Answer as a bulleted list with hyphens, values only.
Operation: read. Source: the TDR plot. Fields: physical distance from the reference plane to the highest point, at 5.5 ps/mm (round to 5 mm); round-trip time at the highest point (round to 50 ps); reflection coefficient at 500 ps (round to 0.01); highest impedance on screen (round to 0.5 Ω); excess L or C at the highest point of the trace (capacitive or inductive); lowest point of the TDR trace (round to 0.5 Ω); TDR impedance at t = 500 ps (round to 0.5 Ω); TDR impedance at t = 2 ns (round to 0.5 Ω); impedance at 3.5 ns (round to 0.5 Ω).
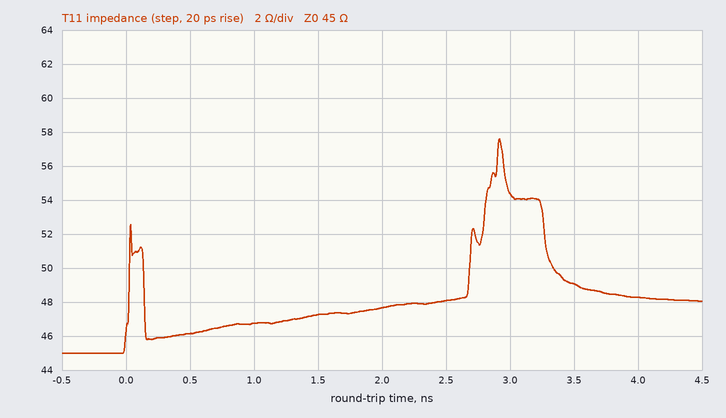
- 265 mm
- 2.90 ns
- +0.01
- 57.5 Ω
- inductive
- 45.0 Ω
- 46.0 Ω
- 47.5 Ω
- 49.0 Ω
